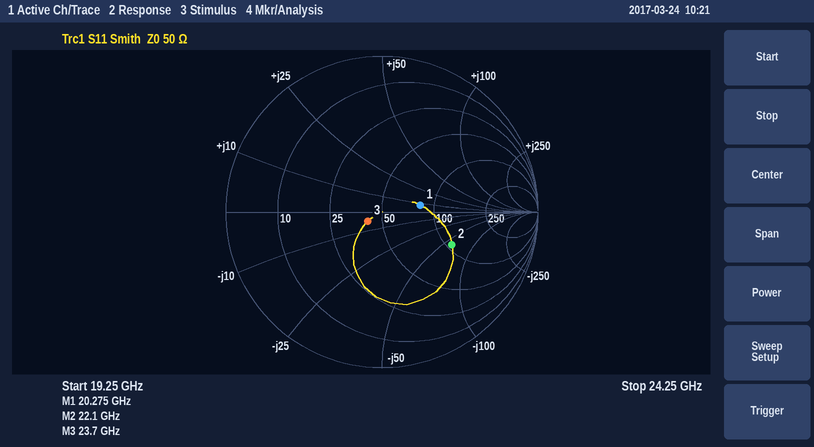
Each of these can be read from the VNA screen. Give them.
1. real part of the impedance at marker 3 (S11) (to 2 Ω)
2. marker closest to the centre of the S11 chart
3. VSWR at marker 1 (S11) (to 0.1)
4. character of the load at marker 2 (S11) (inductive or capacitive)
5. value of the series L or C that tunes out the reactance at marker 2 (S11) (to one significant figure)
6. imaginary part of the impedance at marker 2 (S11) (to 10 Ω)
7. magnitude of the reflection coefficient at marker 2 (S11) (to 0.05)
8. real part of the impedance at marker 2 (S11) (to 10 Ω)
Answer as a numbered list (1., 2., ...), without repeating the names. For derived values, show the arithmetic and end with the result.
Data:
1. 42 Ω
2. marker 3
3. 1.7
4. capacitive
5. L = 60 Ω/(2π × 22.1 GHz) ≈ 432 pH, so 400 pH to one significant figure
6. -60 Ω
7. 0.50
8. 110 Ω
